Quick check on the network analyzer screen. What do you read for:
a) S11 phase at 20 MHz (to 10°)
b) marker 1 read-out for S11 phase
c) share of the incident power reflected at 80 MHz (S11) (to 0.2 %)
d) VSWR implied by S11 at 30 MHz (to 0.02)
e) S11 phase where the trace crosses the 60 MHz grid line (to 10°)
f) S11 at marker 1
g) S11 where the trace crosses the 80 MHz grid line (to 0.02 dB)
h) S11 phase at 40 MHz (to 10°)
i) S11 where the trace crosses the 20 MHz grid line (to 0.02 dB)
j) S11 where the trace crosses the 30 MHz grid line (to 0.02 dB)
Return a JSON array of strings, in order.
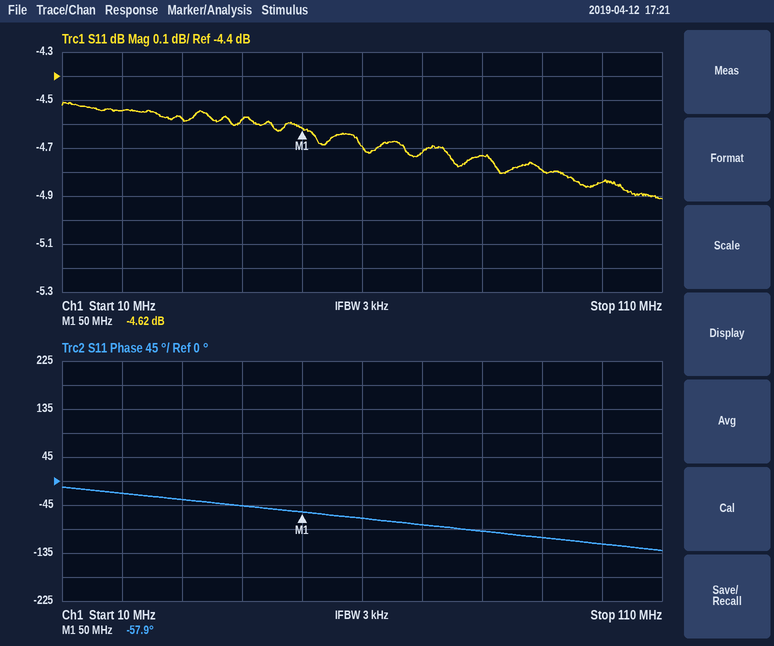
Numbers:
["-20°", "-57.9°", "33.6 %", "3.88", "-70°", "-4.62 dB", "-4.74 dB", "-50°", "-4.54 dB", "-4.58 dB"]
